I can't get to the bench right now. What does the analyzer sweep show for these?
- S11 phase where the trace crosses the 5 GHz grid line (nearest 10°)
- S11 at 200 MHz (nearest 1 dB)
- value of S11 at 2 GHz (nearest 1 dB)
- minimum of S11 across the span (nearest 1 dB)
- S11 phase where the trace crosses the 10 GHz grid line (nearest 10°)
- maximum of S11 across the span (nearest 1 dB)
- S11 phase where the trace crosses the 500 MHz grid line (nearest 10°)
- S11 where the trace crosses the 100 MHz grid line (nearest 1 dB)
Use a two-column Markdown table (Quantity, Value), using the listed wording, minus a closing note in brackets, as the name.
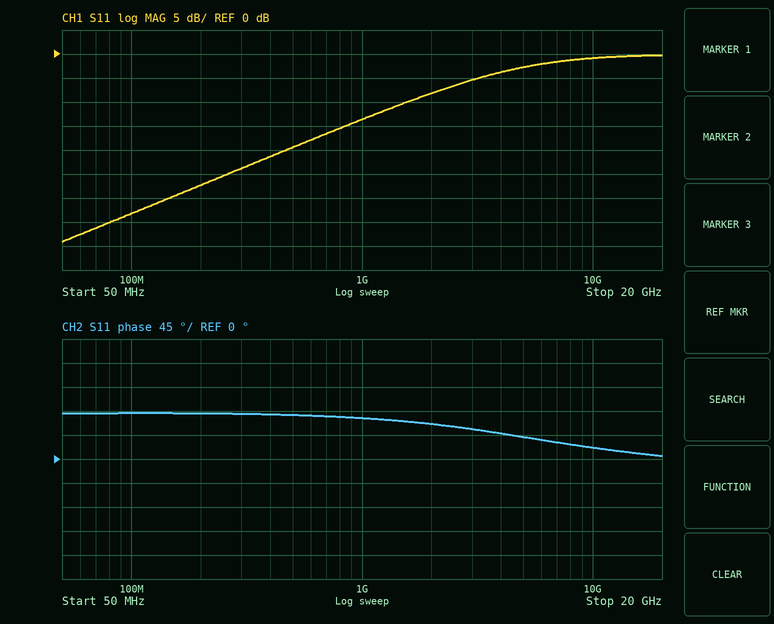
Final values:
| Quantity | Value |
|---|---|
| S11 phase where the trace crosses the 5 GHz grid line | 40° |
| S11 at 200 MHz | -27 dB |
| value of S11 at 2 GHz | -8 dB |
| minimum of S11 across the span | -39 dB |
| S11 phase where the trace crosses the 10 GHz grid line | 20° |
| maximum of S11 across the span | 0 dB |
| S11 phase where the trace crosses the 500 MHz grid line | 80° |
| S11 where the trace crosses the 100 MHz grid line | -33 dB |
